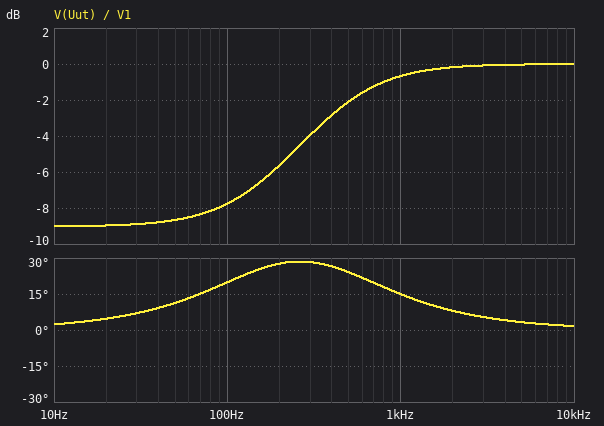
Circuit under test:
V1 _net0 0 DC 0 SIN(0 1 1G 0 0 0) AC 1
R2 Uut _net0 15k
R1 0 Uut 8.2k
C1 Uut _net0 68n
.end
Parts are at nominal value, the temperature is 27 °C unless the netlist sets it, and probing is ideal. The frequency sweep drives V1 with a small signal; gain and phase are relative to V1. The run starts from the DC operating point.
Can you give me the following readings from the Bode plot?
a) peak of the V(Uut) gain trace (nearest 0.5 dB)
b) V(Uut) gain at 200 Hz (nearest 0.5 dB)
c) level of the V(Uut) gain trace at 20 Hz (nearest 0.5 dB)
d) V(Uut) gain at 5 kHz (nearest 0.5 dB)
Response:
0 dB
-5.5 dB
-9.0 dB
0 dB
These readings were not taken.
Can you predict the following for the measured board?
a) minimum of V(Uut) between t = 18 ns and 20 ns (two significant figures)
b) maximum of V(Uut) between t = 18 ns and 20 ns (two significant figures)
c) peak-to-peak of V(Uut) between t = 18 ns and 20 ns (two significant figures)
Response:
-1.0 V
1.0 V
2.0 V
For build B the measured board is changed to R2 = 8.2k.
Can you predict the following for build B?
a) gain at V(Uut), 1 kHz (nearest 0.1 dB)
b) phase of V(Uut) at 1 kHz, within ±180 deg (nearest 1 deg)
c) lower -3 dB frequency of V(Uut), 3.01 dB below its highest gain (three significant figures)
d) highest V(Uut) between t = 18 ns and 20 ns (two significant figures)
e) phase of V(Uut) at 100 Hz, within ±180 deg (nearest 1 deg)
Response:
-0.9 dB
14 deg
404 Hz
1.0 V
9 deg
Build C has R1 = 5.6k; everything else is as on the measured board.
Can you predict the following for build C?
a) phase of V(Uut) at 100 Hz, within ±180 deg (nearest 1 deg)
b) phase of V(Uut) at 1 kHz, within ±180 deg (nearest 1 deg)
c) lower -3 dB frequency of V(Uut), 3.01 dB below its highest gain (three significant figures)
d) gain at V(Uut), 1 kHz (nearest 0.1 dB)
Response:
23 deg
21 deg
530 Hz
-1.1 dB
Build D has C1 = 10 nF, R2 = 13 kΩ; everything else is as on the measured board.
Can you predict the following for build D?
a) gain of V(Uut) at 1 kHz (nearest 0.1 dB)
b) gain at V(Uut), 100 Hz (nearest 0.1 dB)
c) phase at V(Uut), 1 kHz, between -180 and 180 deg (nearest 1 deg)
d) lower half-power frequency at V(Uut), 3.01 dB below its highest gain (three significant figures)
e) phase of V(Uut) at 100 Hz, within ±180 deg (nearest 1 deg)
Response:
-6.4 dB
-8.2 dB
22 deg
2.65 kHz
3 deg
